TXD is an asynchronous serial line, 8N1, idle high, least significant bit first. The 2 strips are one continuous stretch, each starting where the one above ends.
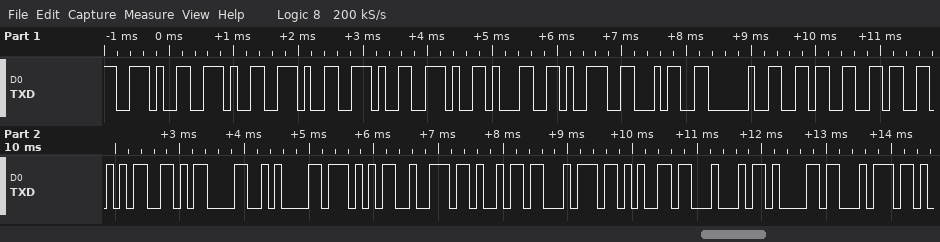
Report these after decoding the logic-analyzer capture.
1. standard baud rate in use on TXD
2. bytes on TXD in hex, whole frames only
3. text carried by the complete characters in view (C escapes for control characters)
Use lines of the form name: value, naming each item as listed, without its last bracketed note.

standard baud rate in use on TXD: 9600 baud
bytes on TXD in hex, whole frames only: 2E 2E 2E 2E 2E 31 39 34 20 36 36 35 0D 0A 57 72 69 74 65 44 61 74
text carried by the complete characters in view: ".....194 665\r\nWriteDat"
